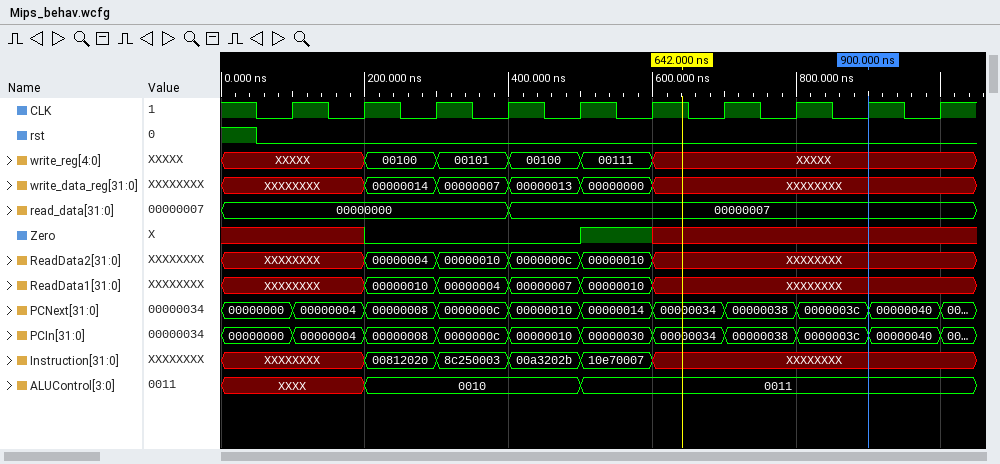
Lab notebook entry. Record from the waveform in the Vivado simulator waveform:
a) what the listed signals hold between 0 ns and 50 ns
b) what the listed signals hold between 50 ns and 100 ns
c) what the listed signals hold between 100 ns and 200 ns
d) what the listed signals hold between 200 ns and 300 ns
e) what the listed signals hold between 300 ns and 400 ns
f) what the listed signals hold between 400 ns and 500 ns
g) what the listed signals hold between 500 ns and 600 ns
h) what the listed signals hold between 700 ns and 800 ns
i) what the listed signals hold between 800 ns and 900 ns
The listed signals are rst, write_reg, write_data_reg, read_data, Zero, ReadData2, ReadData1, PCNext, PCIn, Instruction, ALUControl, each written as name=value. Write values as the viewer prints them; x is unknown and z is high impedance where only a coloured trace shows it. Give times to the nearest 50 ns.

rst=1, write_reg=XXXXX, write_data_reg=XXXXXXXX, read_data=00000000, Zero=x, ReadData2=XXXXXXXX, ReadData1=XXXXXXXX, PCNext=00000000, PCIn=00000000, Instruction=XXXXXXXX, ALUControl=XXXX
rst=0, write_reg=XXXXX, write_data_reg=XXXXXXXX, read_data=00000000, Zero=x, ReadData2=XXXXXXXX, ReadData1=XXXXXXXX, PCNext=00000000, PCIn=00000000, Instruction=XXXXXXXX, ALUControl=XXXX
rst=0, write_reg=XXXXX, write_data_reg=XXXXXXXX, read_data=00000000, Zero=x, ReadData2=XXXXXXXX, ReadData1=XXXXXXXX, PCNext=00000004, PCIn=00000004, Instruction=XXXXXXXX, ALUControl=XXXX
rst=0, write_reg=00100, write_data_reg=00000014, read_data=00000000, Zero=0, ReadData2=00000004, ReadData1=00000010, PCNext=00000008, PCIn=00000008, Instruction=00812020, ALUControl=0010
rst=0, write_reg=00101, write_data_reg=00000007, read_data=00000000, Zero=0, ReadData2=00000010, ReadData1=00000004, PCNext=0000000c, PCIn=0000000c, Instruction=8c250003, ALUControl=0010
rst=0, write_reg=00100, write_data_reg=00000013, read_data=00000007, Zero=0, ReadData2=0000000c, ReadData1=00000007, PCNext=00000010, PCIn=00000010, Instruction=00a3202b, ALUControl=0010
rst=0, write_reg=00111, write_data_reg=00000000, read_data=00000007, Zero=1, ReadData2=00000010, ReadData1=00000010, PCNext=00000014, PCIn=00000030, Instruction=10e70007, ALUControl=0011
rst=0, write_reg=XXXXX, write_data_reg=XXXXXXXX, read_data=00000007, Zero=x, ReadData2=XXXXXXXX, ReadData1=XXXXXXXX, PCNext=00000038, PCIn=00000038, Instruction=XXXXXXXX, ALUControl=0011
rst=0, write_reg=XXXXX, write_data_reg=XXXXXXXX, read_data=00000007, Zero=x, ReadData2=XXXXXXXX, ReadData1=XXXXXXXX, PCNext=0000003c, PCIn=0000003c, Instruction=XXXXXXXX, ALUControl=0011
